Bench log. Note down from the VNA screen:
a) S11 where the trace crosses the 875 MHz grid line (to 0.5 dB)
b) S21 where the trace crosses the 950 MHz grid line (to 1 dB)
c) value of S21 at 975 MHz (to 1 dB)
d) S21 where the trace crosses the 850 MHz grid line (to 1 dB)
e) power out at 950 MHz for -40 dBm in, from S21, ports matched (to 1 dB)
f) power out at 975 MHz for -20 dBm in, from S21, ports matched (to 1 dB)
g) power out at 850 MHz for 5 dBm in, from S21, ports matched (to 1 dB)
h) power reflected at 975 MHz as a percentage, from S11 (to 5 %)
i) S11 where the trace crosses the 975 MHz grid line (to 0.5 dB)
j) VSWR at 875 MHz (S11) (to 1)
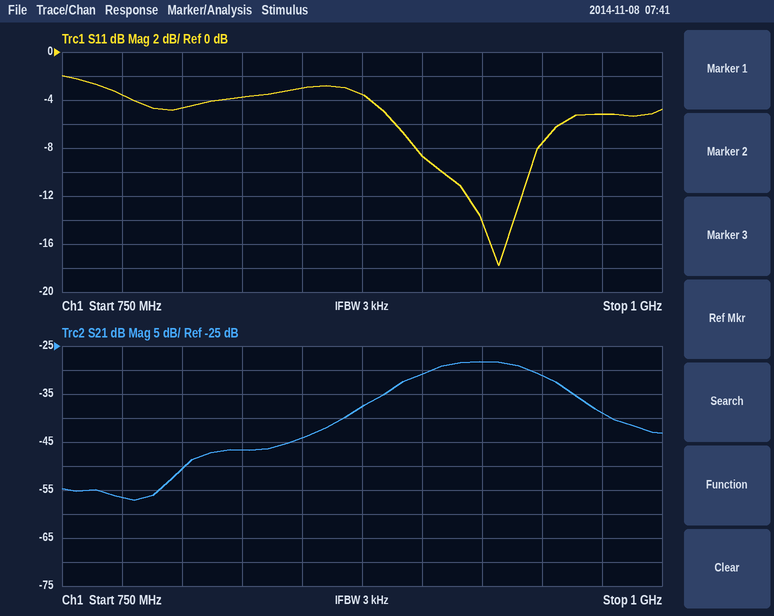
-3.5 dB
-31 dB
-39 dB
-44 dB
-71 dBm
-59 dBm
-39 dBm
30 %
-5.0 dB
5
